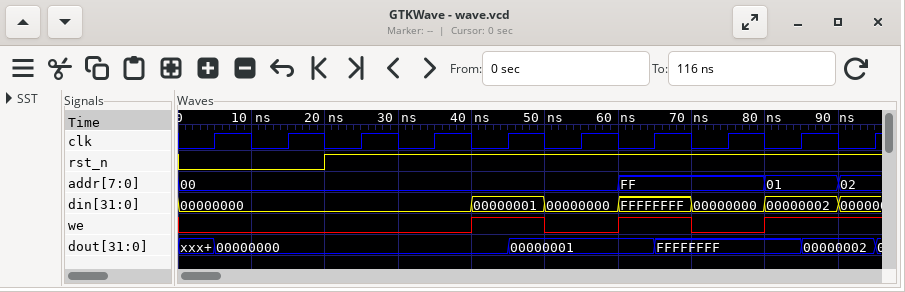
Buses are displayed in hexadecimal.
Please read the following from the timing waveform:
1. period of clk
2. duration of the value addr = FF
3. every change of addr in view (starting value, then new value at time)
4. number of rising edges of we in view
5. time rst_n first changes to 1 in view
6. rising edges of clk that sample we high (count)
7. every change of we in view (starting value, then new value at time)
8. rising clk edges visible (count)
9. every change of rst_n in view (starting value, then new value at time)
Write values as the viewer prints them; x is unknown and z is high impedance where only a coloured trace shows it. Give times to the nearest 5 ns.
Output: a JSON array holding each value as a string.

["10 ns", "20 ns", "00, FF at 60 ns, 01 at 80 ns, 02 at 90 ns", "3", "20 ns", "4", "0, 1 at 40 ns, 0 at 50 ns, 1 at 60 ns, 0 at 70 ns, 1 at 80 ns", "10", "0, 1 at 20 ns"]
